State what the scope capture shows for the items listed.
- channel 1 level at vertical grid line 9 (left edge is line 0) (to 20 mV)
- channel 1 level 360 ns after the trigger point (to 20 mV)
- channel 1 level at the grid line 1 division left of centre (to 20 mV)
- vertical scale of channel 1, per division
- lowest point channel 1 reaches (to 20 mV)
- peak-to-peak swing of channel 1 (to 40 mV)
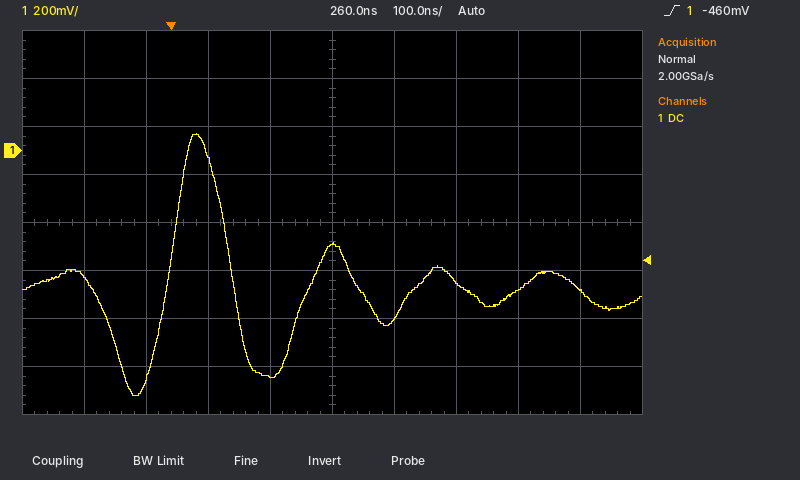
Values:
-580 mV
-700 mV
-940 mV
200 mV
-1.02 V
1.08 V
